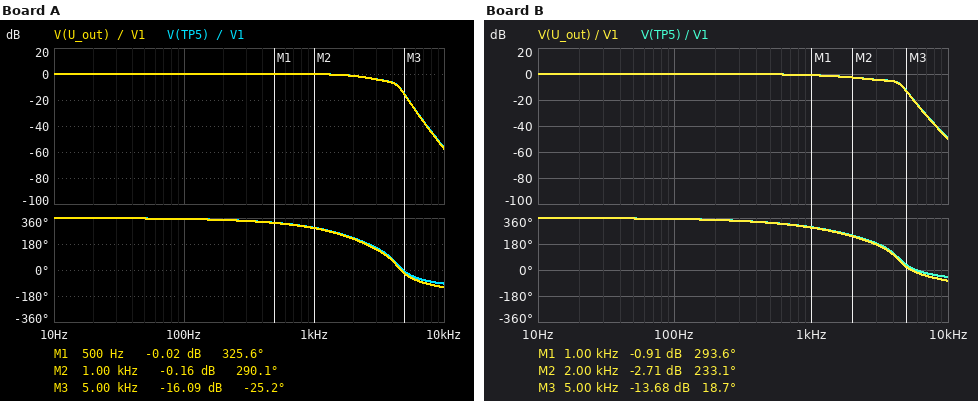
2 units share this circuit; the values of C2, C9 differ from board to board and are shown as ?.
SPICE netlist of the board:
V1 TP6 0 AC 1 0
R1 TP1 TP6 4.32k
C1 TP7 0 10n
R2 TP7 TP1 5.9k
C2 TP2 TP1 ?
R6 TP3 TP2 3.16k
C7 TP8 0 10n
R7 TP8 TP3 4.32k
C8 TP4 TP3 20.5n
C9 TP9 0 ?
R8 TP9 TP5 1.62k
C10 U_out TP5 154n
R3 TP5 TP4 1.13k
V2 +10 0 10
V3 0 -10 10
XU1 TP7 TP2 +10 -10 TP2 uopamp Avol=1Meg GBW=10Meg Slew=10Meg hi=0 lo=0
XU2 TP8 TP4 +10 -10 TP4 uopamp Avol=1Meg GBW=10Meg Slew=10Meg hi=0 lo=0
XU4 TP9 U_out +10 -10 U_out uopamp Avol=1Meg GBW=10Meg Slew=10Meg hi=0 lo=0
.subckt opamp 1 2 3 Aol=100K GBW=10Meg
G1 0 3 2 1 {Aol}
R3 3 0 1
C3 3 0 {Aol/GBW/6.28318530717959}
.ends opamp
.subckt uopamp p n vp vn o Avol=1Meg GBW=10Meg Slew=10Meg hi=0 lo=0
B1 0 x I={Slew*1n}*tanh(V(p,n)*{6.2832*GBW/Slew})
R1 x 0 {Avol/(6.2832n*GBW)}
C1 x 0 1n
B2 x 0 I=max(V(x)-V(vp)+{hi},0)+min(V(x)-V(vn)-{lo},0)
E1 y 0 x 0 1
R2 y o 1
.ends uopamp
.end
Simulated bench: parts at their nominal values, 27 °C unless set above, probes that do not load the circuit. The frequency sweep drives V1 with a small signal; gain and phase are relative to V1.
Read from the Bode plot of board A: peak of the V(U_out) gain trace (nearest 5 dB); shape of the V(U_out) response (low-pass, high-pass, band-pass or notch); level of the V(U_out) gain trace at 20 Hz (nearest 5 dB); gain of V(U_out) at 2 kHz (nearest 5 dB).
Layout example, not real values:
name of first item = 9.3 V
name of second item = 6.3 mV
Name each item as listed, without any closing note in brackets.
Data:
peak of the V(U_out) gain trace = 0 dB
shape of the V(U_out) response = low-pass
level of the V(U_out) gain trace at 20 Hz = 0 dB
gain of V(U_out) at 2 kHz = 0 dB
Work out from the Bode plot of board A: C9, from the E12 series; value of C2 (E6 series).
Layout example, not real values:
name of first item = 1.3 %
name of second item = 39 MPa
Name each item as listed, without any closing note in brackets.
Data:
C9, from the E12 series = 4.7 nF
value of C2 = 15 nF
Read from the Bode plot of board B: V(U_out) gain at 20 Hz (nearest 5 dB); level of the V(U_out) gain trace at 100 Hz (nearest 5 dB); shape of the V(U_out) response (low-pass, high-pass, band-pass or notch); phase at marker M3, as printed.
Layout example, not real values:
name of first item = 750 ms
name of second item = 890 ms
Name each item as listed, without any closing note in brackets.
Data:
V(U_out) gain at 20 Hz = 0 dB
level of the V(U_out) gain trace at 100 Hz = 0 dB
shape of the V(U_out) response = low-pass
phase at marker M3, as printed = 18.7 deg
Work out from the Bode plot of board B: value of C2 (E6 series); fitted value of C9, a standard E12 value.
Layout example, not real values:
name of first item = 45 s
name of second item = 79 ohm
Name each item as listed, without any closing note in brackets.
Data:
value of C2 = 3.3 nF
fitted value of C9, a standard E12 value = 4.7 nF
